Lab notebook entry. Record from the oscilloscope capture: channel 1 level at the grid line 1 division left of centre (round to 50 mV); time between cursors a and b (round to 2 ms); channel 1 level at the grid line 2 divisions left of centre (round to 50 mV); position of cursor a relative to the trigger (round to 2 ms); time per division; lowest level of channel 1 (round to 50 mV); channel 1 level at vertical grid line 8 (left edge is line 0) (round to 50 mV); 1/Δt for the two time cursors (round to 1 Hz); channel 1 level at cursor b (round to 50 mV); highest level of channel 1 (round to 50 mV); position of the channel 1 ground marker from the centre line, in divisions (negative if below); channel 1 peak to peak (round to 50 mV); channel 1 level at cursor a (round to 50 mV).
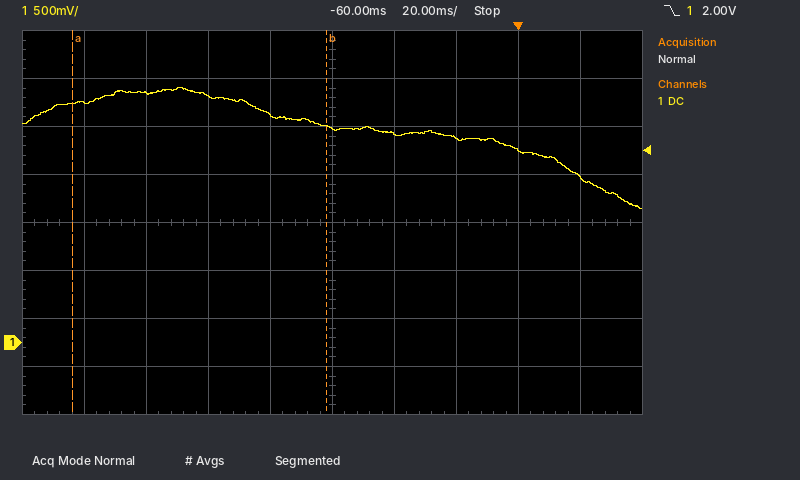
2.35 V
82 ms
2.55 V
-144 ms
20 ms
1.40 V
2.00 V
12 Hz
2.25 V
2.65 V
-2.5 div
1.25 V
2.50 V
